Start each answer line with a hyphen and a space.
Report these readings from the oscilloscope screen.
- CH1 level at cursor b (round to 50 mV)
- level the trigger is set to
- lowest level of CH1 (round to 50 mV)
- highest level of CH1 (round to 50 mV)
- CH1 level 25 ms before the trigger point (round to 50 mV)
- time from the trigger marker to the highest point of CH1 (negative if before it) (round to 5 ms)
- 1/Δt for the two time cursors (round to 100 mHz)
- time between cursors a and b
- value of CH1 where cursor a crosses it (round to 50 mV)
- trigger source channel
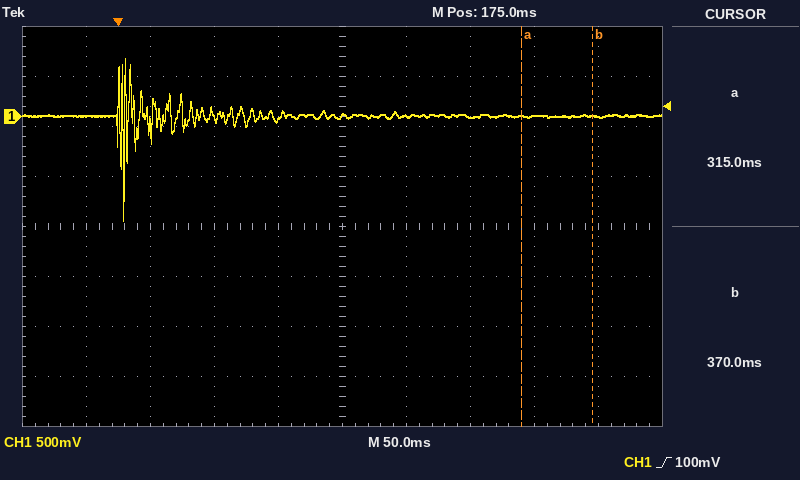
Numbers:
- 0 mV
- 100 mV
- -1.05 V
- 600 mV
- 0 mV
- +5 ms
- 18.2 Hz
- 55 ms
- 0 mV
- CH1
